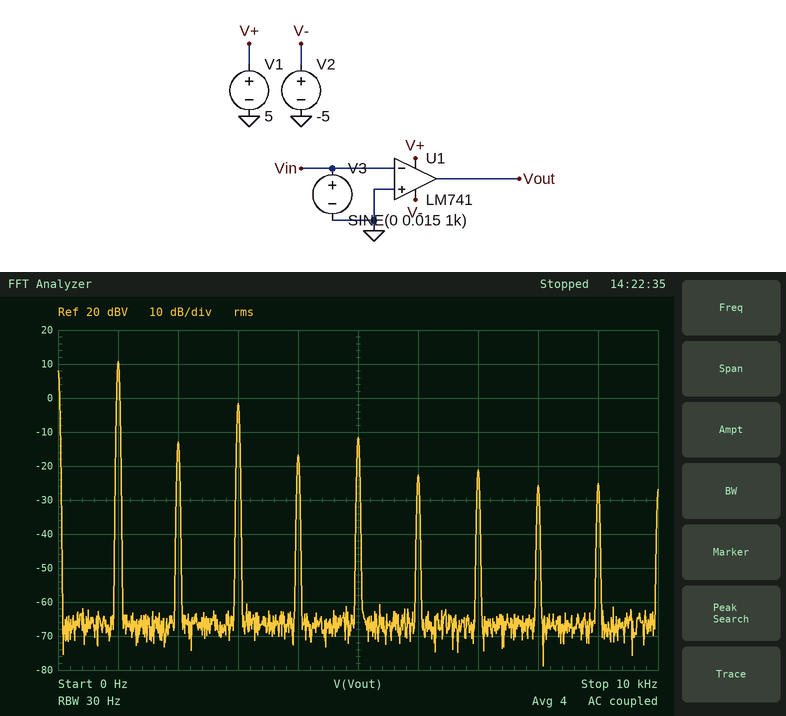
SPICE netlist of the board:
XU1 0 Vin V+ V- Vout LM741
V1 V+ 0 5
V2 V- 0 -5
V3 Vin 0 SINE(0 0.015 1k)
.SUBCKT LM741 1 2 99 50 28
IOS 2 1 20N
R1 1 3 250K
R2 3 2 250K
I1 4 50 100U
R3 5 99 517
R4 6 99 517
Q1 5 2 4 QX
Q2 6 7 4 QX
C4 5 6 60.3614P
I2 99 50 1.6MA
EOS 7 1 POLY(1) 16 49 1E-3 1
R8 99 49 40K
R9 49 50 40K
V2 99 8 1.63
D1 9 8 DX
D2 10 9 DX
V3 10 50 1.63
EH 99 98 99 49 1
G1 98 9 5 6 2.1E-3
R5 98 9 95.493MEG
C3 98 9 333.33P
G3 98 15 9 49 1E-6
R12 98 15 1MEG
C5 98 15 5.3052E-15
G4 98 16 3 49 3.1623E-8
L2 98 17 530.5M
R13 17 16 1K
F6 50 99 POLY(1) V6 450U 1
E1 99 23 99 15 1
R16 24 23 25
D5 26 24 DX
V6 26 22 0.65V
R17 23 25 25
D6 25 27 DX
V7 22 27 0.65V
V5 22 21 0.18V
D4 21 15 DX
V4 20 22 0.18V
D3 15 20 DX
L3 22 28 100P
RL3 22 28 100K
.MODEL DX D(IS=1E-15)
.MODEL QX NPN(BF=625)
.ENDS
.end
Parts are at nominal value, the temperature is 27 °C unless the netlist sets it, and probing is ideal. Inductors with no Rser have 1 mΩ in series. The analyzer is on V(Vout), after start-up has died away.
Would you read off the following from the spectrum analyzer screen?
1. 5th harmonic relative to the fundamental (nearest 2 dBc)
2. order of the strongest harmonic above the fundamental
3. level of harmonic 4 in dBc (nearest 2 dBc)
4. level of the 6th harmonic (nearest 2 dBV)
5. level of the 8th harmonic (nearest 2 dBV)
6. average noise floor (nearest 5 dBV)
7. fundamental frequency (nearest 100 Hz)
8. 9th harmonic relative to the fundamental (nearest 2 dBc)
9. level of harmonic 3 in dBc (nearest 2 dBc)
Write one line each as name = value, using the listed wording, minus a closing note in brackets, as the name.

5th harmonic relative to the fundamental = -22 dBc
order of the strongest harmonic above the fundamental = 3
level of harmonic 4 in dBc = -28 dBc
level of the 6th harmonic = -22 dBV
level of the 8th harmonic = -26 dBV
average noise floor = -65 dBV
fundamental frequency = 1.0 kHz
9th harmonic relative to the fundamental = -36 dBc
level of harmonic 3 in dBc = -12 dBc
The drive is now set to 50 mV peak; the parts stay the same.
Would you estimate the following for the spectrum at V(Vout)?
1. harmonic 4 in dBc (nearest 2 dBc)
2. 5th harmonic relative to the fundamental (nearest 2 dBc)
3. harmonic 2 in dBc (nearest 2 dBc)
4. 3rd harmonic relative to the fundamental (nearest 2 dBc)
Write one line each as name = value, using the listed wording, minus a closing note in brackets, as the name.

harmonic 4 in dBc = -36 dBc
5th harmonic relative to the fundamental = -16 dBc
harmonic 2 in dBc = -34 dBc
3rd harmonic relative to the fundamental = -10 dBc
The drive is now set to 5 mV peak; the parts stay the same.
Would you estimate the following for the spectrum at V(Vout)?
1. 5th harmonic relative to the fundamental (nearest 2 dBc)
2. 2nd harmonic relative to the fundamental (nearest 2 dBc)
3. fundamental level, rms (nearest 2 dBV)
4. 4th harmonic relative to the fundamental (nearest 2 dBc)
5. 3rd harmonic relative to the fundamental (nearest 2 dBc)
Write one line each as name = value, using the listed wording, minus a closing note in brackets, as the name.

5th harmonic relative to the fundamental = -34 dBc
2nd harmonic relative to the fundamental = -14 dBc
fundamental level, rms = 8 dBV
4th harmonic relative to the fundamental = -30 dBc
3rd harmonic relative to the fundamental = -22 dBc
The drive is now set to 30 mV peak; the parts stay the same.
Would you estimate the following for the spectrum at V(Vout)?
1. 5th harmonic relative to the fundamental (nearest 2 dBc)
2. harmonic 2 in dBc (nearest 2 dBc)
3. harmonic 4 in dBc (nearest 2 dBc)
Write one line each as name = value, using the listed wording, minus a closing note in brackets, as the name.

5th harmonic relative to the fundamental = -18 dBc
harmonic 2 in dBc = -30 dBc
harmonic 4 in dBc = -32 dBc
